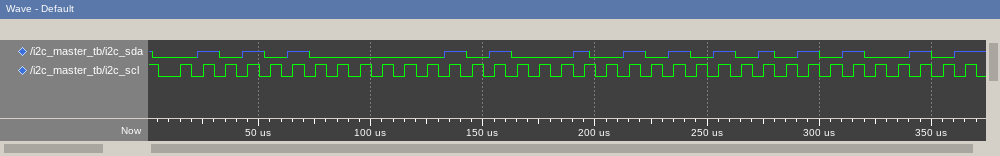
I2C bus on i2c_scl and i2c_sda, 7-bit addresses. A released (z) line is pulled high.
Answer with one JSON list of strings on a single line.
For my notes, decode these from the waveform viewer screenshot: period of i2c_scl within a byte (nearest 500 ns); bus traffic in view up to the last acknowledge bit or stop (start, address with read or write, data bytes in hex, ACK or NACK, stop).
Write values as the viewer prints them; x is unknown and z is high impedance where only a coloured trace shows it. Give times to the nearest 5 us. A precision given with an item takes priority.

["10000 ns", "start, address 2A write ACK, 14 ACK, repeated start, address 2A read ACK"]
